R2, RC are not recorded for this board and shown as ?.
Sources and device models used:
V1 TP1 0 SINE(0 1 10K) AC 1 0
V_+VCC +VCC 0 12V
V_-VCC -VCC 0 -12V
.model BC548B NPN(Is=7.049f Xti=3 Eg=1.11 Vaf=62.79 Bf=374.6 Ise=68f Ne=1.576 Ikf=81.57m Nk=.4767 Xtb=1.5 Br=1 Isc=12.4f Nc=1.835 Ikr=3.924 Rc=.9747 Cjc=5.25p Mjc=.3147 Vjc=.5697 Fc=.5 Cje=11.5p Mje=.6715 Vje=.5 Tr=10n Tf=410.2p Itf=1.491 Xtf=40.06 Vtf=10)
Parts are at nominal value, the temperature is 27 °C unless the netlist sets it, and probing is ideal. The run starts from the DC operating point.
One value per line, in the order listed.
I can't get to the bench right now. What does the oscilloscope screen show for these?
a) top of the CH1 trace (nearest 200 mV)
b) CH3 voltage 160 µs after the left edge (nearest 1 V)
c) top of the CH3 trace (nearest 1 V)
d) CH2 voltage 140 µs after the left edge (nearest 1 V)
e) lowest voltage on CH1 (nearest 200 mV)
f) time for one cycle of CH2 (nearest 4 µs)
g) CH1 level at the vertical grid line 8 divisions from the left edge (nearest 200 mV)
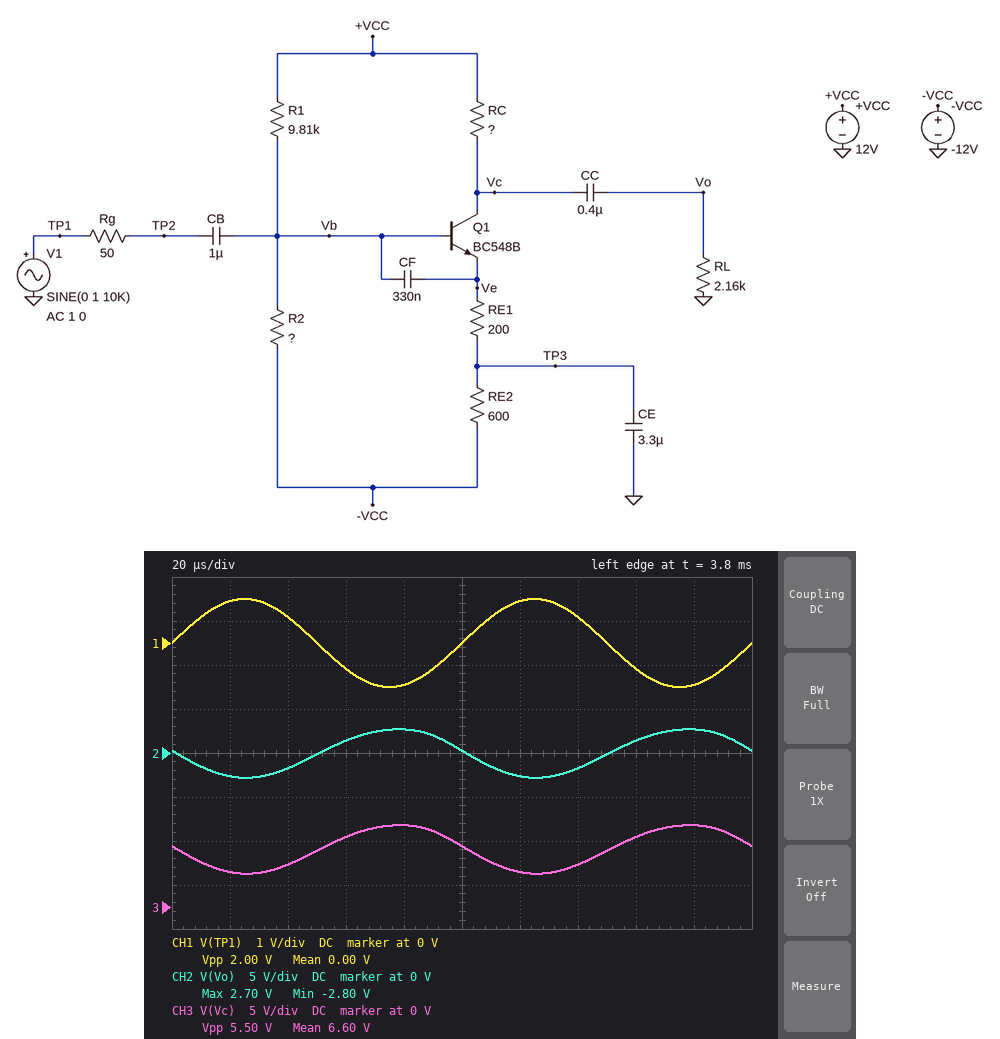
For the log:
1.0 V
8 V
9 V
-2 V
-1.0 V
100 µs
-600 mV
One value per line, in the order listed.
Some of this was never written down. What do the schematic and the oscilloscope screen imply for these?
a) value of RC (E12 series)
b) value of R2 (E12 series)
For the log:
820 Ω
3.3 kΩ
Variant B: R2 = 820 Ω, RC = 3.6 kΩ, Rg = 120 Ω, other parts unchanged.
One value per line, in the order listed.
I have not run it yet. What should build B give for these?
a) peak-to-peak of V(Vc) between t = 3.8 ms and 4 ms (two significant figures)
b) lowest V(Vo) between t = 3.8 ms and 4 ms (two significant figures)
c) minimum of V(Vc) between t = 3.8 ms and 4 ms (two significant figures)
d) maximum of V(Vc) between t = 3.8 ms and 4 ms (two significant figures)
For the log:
6.9 V
-4.9 V
1.7 V
8.6 V
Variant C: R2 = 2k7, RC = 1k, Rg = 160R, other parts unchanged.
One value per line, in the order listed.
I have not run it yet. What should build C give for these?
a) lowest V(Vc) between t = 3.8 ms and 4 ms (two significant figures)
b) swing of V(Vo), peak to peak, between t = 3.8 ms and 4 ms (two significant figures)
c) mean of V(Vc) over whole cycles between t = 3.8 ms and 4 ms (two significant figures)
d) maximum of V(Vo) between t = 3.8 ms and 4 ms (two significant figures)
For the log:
3.4 V
5.8 V
6.5 V
2.8 V
